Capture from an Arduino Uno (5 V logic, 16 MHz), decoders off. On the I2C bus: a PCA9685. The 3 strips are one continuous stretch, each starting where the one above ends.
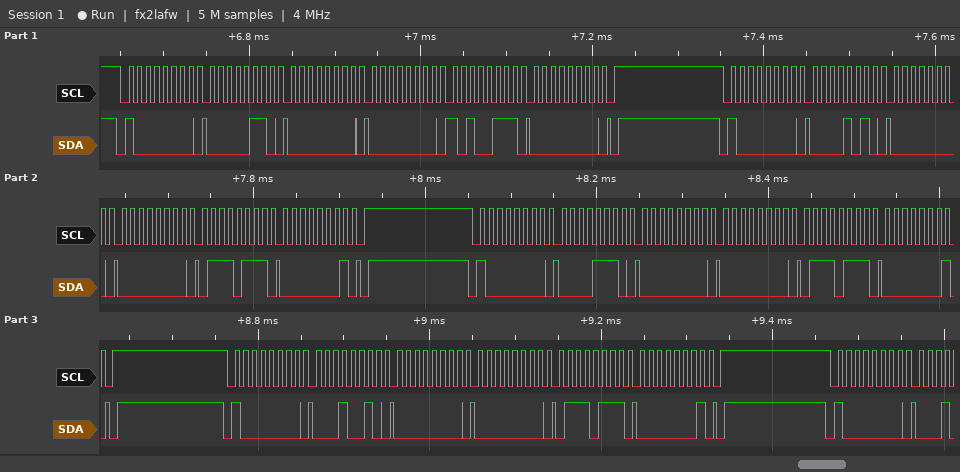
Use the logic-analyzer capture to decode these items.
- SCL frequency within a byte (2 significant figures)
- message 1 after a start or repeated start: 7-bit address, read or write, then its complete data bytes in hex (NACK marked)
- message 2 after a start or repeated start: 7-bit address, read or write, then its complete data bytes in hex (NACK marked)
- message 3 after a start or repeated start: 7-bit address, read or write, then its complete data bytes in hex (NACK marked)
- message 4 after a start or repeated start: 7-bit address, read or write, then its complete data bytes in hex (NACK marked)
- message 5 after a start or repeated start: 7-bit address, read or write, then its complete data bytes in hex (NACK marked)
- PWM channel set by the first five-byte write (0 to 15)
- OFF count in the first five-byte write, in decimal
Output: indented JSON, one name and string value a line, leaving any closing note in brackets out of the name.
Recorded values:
{
  "SCL frequency within a byte": "100 kHz",
  "message 1 after a start or repeated start: 7-bit address, read or write, then its complete data bytes in hex": "0x40 write: 06 00 00 A7 00",
  "message 2 after a start or repeated start: 7-bit address, read or write, then its complete data bytes in hex": "0x40 write: 0A 00 00 77 01",
  "message 3 after a start or repeated start: 7-bit address, read or write, then its complete data bytes in hex": "0x40 write: 0E 00 00 77 01",
  "message 4 after a start or repeated start: 7-bit address, read or write, then its complete data bytes in hex": "0x40 write: 12 00 00 77 01",
  "message 5 after a start or repeated start: 7-bit address, read or write, then its complete data bytes in hex": "0x40 write",
  "PWM channel set by the first five-byte write": "0",
  "OFF count in the first five-byte write, in decimal": "167"
}
